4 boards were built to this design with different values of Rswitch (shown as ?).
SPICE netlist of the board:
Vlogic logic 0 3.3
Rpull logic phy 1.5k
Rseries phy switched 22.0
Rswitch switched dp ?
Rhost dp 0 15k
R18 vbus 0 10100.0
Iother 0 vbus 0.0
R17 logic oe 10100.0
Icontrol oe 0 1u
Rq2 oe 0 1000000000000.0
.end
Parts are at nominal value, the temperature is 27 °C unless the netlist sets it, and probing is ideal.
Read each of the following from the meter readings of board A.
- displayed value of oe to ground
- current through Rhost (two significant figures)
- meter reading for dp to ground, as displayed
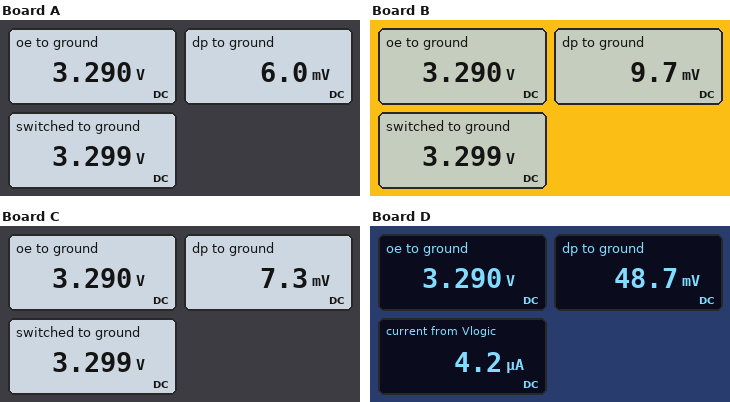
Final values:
3.290 V
400 nA
6.0 mV
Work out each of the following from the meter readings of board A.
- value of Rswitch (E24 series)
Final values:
8.2 MΩ
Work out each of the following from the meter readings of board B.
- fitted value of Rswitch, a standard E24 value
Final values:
5.1 MΩ
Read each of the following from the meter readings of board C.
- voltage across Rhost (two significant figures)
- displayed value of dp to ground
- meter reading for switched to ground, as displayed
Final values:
7.3 mV
7.3 mV
3.299 V
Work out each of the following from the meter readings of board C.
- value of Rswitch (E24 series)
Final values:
6.8 MΩ
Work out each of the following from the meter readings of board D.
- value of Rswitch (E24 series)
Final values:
1 MΩ
